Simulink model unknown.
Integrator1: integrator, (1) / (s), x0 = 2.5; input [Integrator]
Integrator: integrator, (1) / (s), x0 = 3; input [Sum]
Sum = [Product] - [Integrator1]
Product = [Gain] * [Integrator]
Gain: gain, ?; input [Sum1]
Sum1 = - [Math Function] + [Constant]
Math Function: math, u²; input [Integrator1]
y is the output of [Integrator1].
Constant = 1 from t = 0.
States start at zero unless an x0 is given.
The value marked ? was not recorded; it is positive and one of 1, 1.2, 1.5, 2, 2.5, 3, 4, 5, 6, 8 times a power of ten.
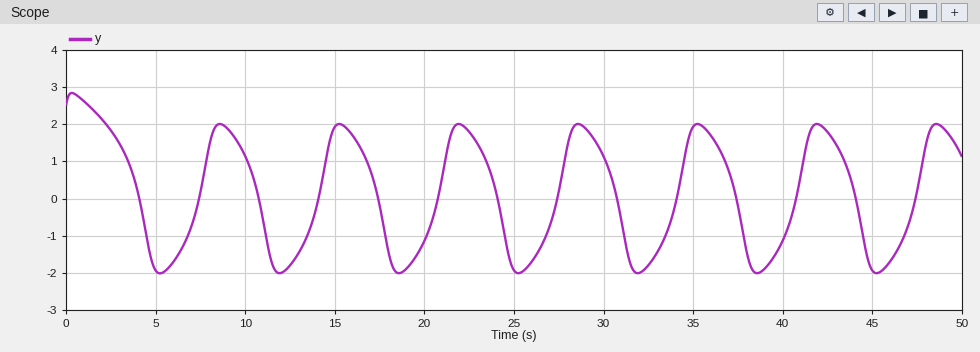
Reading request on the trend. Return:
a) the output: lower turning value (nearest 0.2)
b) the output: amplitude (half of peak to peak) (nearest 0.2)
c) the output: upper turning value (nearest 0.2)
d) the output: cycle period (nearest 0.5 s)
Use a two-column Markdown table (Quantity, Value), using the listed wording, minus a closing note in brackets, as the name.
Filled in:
| Quantity | Value |
|---|---|
| the output: lower turning value | -2.0 |
| the output: amplitude (half of peak to peak) | 2.0 |
| the output: upper turning value | 2.0 |
| the output: cycle period | 6.5 s |
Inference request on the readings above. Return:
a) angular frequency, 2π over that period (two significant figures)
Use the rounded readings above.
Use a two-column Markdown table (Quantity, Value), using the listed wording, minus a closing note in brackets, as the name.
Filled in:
| Quantity | Value |
|---|---|
| angular frequency, 2π over that period | 0.97 rad/s |
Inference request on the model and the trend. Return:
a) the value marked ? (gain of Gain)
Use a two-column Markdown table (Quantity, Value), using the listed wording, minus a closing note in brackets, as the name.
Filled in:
| Quantity | Value |
|---|---|
| the value marked ? | 1 |
